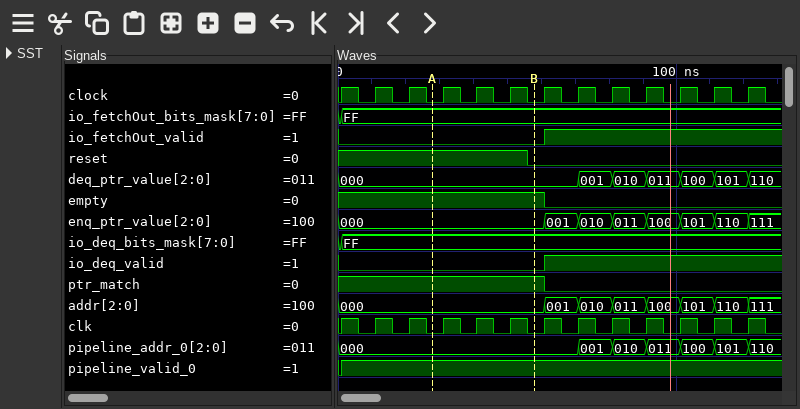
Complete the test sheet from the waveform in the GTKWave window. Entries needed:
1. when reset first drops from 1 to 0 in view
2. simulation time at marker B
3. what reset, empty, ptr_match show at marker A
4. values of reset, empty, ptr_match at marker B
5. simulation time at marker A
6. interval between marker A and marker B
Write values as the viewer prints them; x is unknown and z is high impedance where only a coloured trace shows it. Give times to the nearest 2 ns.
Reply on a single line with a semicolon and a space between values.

56 ns; 58 ns; reset=1, empty=1, ptr_match=1; reset=0, empty=1, ptr_match=1; 28 ns; 30 ns
